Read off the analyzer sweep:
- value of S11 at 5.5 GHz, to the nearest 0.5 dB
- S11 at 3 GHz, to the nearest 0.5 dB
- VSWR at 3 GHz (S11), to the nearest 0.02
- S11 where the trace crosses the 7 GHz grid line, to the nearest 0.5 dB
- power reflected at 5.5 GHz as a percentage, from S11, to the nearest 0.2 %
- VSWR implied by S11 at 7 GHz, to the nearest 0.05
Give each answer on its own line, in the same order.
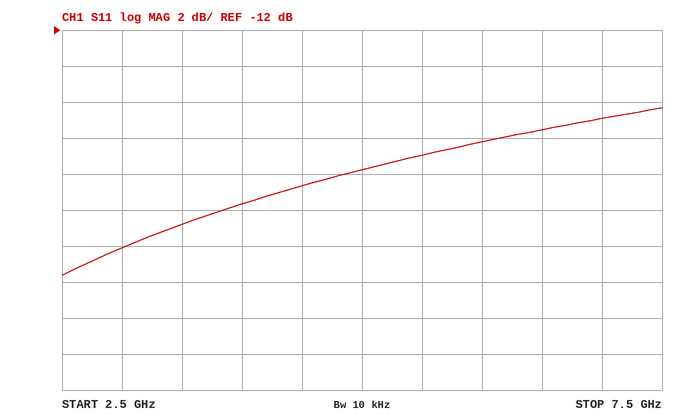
-19.0 dB
-24.0 dB
1.14
-17.0 dB
1.2 %
1.35
